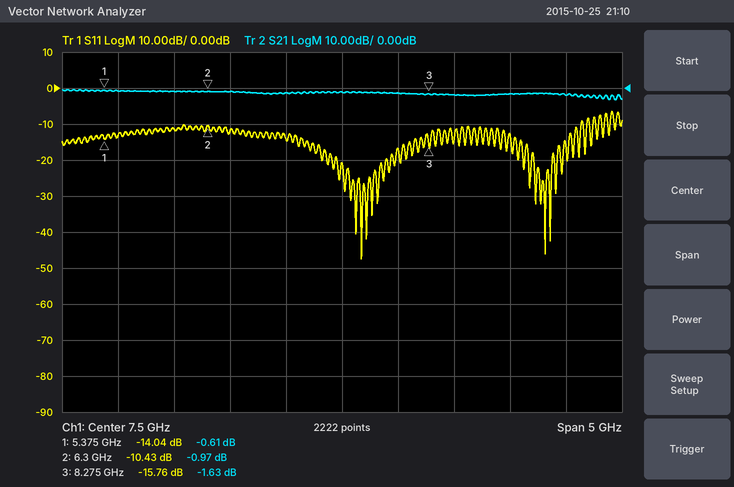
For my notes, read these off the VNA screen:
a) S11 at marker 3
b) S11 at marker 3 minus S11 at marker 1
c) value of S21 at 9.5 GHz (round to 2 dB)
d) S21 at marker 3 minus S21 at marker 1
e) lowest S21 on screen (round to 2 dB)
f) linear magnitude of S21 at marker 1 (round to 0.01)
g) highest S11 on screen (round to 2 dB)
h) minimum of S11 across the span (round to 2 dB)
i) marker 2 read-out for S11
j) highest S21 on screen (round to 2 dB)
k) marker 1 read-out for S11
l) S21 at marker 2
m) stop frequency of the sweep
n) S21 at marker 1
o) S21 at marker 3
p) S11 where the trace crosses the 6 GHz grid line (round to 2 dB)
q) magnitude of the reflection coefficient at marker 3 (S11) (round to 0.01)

-15.76 dB
-1.72 dB
-2 dB
-1.02 dB
-4 dB
0.93
-6 dB
-48 dB
-10.43 dB
0 dB
-14.04 dB
-0.97 dB
10 GHz
-0.61 dB
-1.63 dB
-12 dB
0.16
